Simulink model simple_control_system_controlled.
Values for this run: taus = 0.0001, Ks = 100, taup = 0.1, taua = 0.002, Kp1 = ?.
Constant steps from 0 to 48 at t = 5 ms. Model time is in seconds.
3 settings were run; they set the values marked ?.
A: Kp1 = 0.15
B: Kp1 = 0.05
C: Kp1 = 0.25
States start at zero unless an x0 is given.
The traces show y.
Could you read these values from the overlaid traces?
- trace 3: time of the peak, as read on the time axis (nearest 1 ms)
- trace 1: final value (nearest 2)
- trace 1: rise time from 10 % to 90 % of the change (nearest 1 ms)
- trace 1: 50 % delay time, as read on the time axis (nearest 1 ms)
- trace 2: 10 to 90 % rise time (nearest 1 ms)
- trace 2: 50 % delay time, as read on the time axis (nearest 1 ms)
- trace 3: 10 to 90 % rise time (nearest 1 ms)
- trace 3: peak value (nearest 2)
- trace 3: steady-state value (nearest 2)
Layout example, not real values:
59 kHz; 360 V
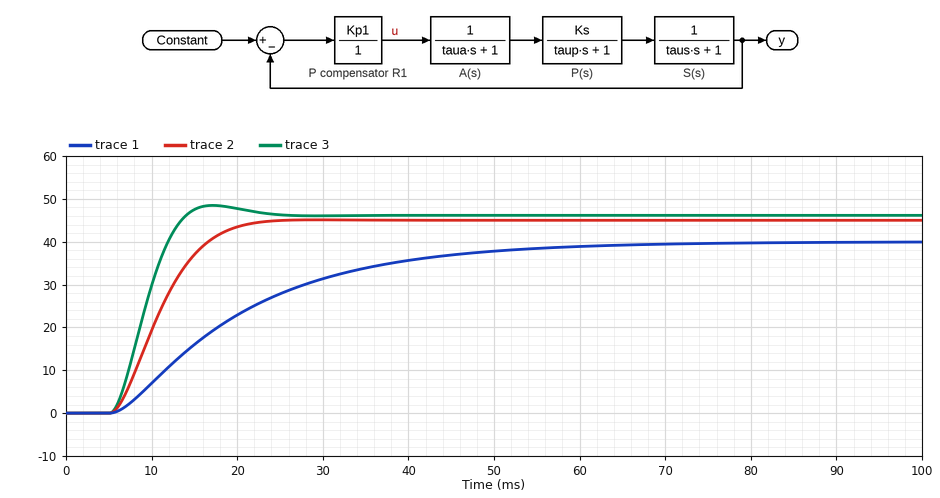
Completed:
17 ms; 40; 33 ms; 18 ms; 10 ms; 11 ms; 6 ms; 48; 46
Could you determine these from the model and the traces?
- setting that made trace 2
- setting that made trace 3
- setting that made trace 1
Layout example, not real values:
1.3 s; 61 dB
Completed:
A; C; B
